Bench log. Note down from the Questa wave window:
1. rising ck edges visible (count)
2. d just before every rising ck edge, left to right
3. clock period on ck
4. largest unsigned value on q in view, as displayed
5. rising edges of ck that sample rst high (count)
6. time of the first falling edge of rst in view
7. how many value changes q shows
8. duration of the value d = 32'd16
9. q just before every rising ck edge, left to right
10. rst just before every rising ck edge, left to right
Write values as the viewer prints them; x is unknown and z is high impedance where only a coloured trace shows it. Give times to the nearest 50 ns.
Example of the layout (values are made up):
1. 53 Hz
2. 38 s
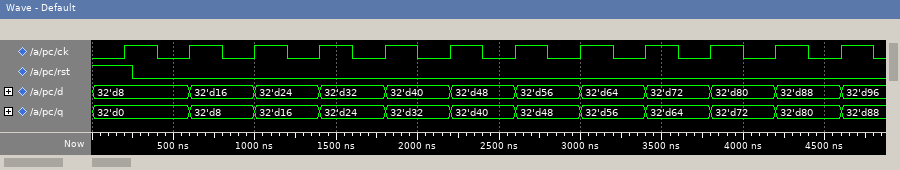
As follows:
1. 12
2. 32'd8, 32'd8, 32'd16, 32'd24, 32'd32, 32'd40, 32'd48, 32'd56, 32'd64, 32'd72, 32'd80, 32'd88
3. 400 ns
4. 32'd88
5. 1
6. 250 ns
7. 11
8. 400 ns
9. 32'd0, 32'd0, 32'd8, 32'd16, 32'd24, 32'd32, 32'd40, 32'd48, 32'd56, 32'd64, 32'd72, 32'd80
10. 1 0 0 0 0 0 0 0 0 0 0 0
